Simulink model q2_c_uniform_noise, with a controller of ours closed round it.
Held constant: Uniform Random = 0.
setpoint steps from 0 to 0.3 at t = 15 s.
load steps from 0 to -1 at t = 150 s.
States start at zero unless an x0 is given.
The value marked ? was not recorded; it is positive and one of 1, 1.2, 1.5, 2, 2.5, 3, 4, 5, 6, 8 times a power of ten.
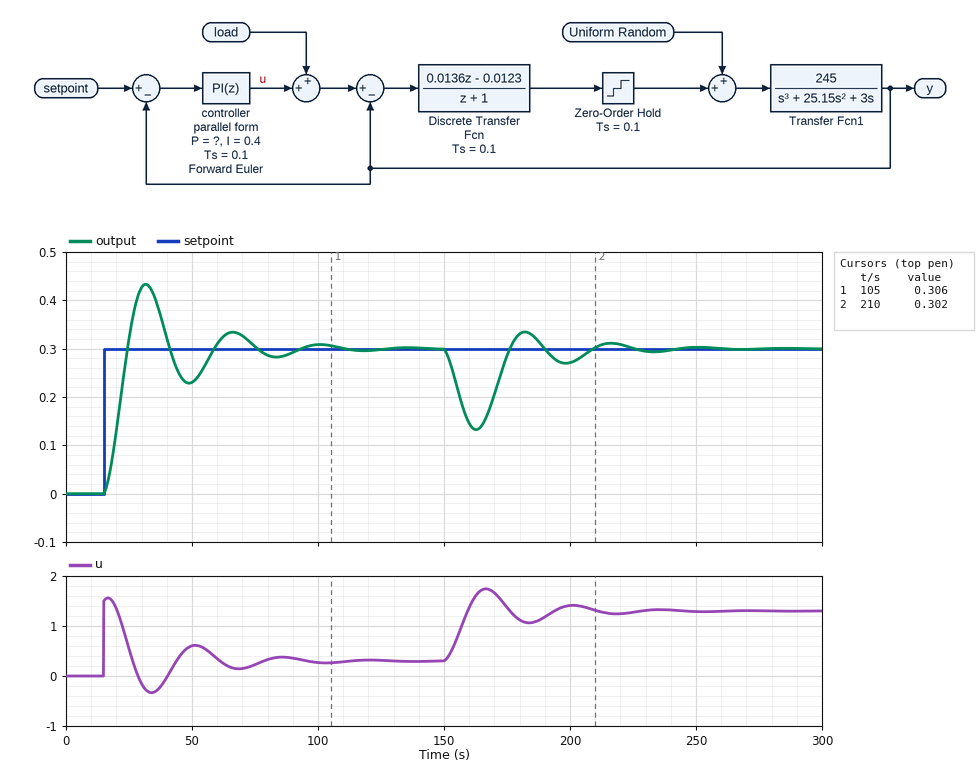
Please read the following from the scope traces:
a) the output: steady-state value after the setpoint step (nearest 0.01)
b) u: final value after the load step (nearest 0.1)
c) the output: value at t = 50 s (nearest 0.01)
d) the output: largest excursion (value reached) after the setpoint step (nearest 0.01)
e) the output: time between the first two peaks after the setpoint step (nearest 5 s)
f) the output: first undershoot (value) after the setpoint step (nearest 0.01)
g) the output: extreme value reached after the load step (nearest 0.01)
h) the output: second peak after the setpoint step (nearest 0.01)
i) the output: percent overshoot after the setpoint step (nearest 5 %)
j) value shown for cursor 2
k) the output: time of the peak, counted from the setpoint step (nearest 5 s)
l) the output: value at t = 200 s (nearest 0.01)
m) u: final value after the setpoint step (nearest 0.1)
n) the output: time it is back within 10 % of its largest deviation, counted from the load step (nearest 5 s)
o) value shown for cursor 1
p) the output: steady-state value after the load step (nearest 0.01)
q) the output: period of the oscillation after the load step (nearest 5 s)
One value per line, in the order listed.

0.30
1.3
0.23
0.43
35 s
0.23
0.13
0.33
45 %
0.302
15 s
0.27
0.3
55 s
0.306
0.30
35 s
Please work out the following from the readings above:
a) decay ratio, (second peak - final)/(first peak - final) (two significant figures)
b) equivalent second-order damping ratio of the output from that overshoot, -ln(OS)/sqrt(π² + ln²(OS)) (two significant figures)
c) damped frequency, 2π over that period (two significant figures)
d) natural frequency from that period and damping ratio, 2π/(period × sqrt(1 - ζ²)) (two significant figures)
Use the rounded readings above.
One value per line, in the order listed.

0.23
0.25
0.18 rad/s
0.19 rad/s
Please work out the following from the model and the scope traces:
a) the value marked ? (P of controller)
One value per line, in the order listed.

5
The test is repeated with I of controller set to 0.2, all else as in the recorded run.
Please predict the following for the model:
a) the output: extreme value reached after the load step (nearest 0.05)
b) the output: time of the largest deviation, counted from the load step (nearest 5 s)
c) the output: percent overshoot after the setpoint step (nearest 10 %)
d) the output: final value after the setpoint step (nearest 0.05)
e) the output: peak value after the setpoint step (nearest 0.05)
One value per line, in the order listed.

0.10
15 s
30 %
0.30
0.40
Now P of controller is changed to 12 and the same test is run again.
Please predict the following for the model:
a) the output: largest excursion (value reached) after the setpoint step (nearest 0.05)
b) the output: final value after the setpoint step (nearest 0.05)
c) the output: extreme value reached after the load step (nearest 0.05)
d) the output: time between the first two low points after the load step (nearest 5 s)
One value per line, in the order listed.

0.40
0.30
0.20
20 s
